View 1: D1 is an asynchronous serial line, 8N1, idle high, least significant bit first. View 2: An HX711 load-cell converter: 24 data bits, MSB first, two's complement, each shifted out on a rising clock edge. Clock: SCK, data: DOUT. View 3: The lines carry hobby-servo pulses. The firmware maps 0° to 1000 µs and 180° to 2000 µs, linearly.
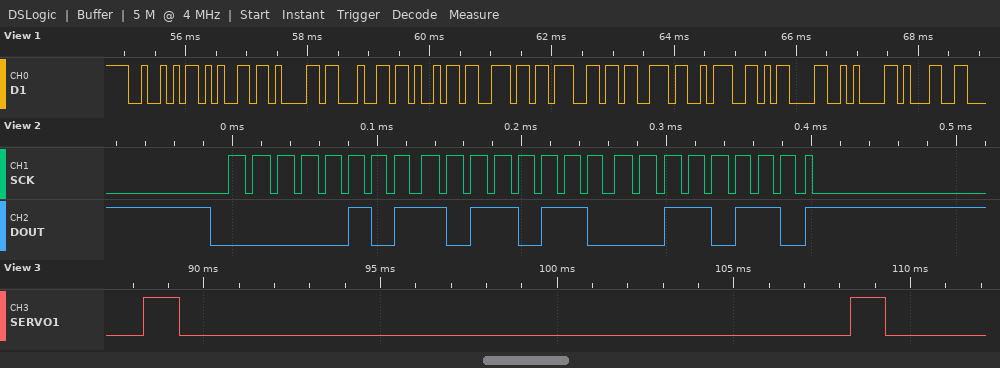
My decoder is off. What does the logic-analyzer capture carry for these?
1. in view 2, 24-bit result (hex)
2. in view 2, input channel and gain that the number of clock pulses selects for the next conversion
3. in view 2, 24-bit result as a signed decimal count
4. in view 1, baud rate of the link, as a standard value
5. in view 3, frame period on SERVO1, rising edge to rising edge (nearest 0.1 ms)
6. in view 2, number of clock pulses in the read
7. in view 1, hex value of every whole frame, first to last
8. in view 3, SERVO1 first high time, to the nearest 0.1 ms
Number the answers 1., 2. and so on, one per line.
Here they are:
1. 0x05B636
2. channel A, gain 128
3. 374326
4. 9600 baud
5. 20.0 ms
6. 25
7. 52 65 61 64 69 6E 67 73 3A 0D 0A 31
8. 1.0 ms
